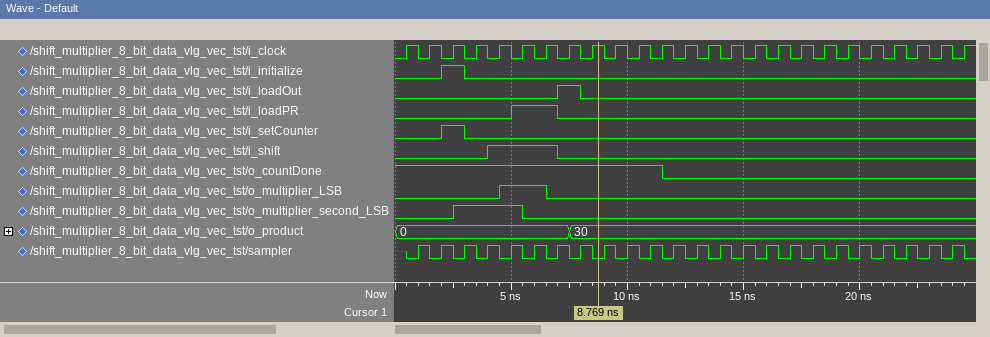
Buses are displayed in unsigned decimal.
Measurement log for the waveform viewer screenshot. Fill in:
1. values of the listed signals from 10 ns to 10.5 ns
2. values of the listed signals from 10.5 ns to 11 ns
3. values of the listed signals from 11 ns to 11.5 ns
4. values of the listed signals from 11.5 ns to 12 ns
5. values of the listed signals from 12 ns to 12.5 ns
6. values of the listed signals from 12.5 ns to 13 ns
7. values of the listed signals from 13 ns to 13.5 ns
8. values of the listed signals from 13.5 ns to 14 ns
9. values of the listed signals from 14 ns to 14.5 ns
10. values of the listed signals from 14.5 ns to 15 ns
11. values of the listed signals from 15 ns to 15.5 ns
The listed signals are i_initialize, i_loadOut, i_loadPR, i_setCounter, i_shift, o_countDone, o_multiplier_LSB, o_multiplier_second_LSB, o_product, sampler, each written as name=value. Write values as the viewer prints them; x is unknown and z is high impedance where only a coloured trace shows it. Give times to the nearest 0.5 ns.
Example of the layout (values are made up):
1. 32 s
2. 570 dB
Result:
1. i_initialize=0, i_loadOut=0, i_loadPR=0, i_setCounter=0, i_shift=0, o_countDone=1, o_multiplier_LSB=0, o_multiplier_second_LSB=0, o_product=30, sampler=1
2. i_initialize=0, i_loadOut=0, i_loadPR=0, i_setCounter=0, i_shift=0, o_countDone=1, o_multiplier_LSB=0, o_multiplier_second_LSB=0, o_product=30, sampler=0
3. i_initialize=0, i_loadOut=0, i_loadPR=0, i_setCounter=0, i_shift=0, o_countDone=1, o_multiplier_LSB=0, o_multiplier_second_LSB=0, o_product=30, sampler=1
4. i_initialize=0, i_loadOut=0, i_loadPR=0, i_setCounter=0, i_shift=0, o_countDone=0, o_multiplier_LSB=0, o_multiplier_second_LSB=0, o_product=30, sampler=0
5. i_initialize=0, i_loadOut=0, i_loadPR=0, i_setCounter=0, i_shift=0, o_countDone=0, o_multiplier_LSB=0, o_multiplier_second_LSB=0, o_product=30, sampler=1
6. i_initialize=0, i_loadOut=0, i_loadPR=0, i_setCounter=0, i_shift=0, o_countDone=0, o_multiplier_LSB=0, o_multiplier_second_LSB=0, o_product=30, sampler=0
7. i_initialize=0, i_loadOut=0, i_loadPR=0, i_setCounter=0, i_shift=0, o_countDone=0, o_multiplier_LSB=0, o_multiplier_second_LSB=0, o_product=30, sampler=1
8. i_initialize=0, i_loadOut=0, i_loadPR=0, i_setCounter=0, i_shift=0, o_countDone=0, o_multiplier_LSB=0, o_multiplier_second_LSB=0, o_product=30, sampler=0
9. i_initialize=0, i_loadOut=0, i_loadPR=0, i_setCounter=0, i_shift=0, o_countDone=0, o_multiplier_LSB=0, o_multiplier_second_LSB=0, o_product=30, sampler=1
10. i_initialize=0, i_loadOut=0, i_loadPR=0, i_setCounter=0, i_shift=0, o_countDone=0, o_multiplier_LSB=0, o_multiplier_second_LSB=0, o_product=30, sampler=0
11. i_initialize=0, i_loadOut=0, i_loadPR=0, i_setCounter=0, i_shift=0, o_countDone=0, o_multiplier_LSB=0, o_multiplier_second_LSB=0, o_product=30, sampler=1
